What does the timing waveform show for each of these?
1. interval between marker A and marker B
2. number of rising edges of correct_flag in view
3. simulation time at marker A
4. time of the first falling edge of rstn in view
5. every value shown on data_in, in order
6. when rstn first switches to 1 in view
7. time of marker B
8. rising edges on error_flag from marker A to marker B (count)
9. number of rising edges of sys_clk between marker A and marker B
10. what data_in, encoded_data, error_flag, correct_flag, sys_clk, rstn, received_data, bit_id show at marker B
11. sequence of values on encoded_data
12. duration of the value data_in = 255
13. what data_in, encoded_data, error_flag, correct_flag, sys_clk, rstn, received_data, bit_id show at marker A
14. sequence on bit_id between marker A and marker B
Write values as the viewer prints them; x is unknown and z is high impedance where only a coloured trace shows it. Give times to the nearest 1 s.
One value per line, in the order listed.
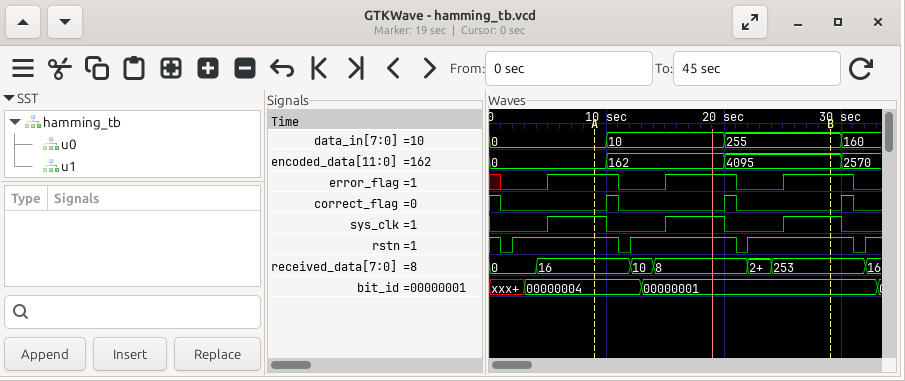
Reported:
20 s
3
9 s
1 s
0, 10, 255, 160
2 s
29 s
2
2
data_in=255, encoded_data=4095, error_flag=1, correct_flag=0, sys_clk=1, rstn=1, received_data=253, bit_id=00000001
0, 162, 4095, 2570
10 s
data_in=0, encoded_data=0, error_flag=1, correct_flag=0, sys_clk=1, rstn=1, received_data=16, bit_id=00000004
00000004, 00000001
